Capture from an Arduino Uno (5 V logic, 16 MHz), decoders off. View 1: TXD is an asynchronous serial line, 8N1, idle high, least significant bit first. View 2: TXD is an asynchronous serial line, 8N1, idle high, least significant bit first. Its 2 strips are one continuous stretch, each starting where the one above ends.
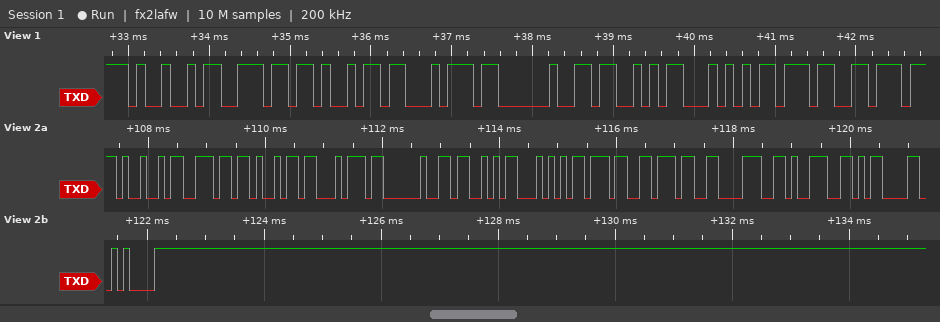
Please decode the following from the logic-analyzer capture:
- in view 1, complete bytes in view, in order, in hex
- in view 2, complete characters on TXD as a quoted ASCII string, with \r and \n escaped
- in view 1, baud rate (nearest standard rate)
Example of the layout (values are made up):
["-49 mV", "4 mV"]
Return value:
["0x49 0x6E 0x69 0x74 0x20 0x53 0x54 0x37", "\"Init ST7789\\r\\n\"", "9600 baud"]
